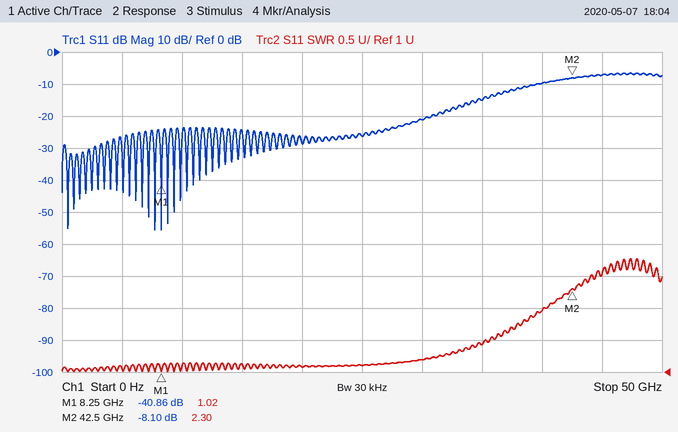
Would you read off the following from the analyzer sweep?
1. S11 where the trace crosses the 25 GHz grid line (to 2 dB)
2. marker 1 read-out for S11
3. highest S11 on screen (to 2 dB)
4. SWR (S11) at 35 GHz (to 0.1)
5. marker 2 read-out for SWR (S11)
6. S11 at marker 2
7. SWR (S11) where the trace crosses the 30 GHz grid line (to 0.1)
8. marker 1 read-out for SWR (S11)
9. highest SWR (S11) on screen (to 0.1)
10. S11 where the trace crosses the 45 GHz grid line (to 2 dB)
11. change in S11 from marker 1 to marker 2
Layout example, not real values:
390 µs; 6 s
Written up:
-26 dB; -40.86 dB; -6 dB; 1.4; 2.30; -8.10 dB; 1.2; 1.02; 2.8; -8 dB; 32.76 dB
